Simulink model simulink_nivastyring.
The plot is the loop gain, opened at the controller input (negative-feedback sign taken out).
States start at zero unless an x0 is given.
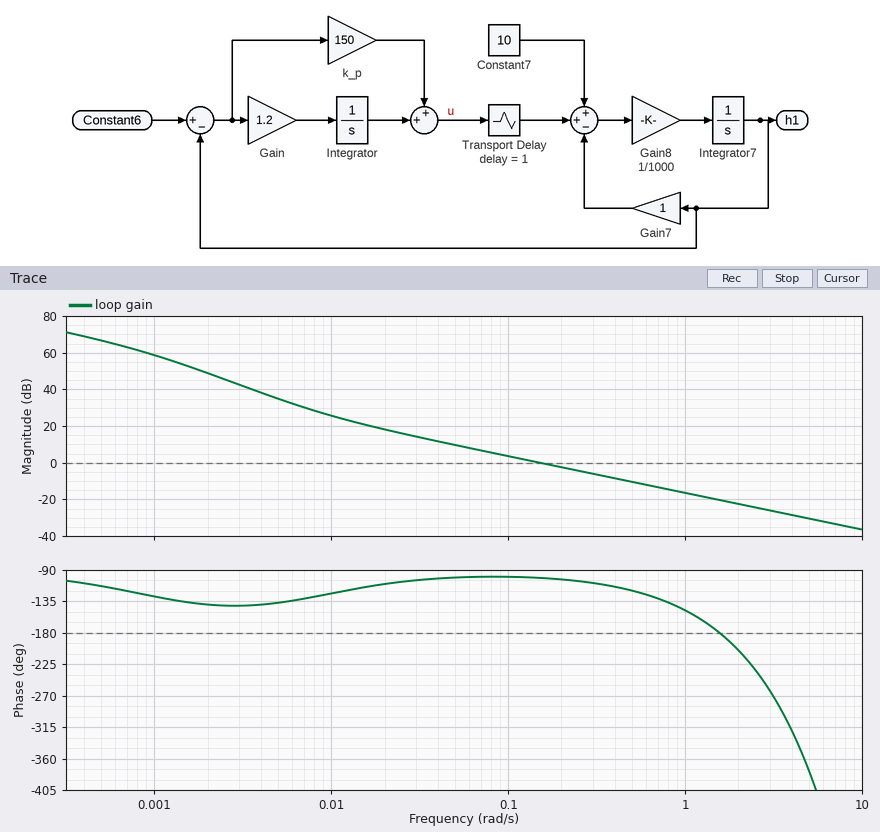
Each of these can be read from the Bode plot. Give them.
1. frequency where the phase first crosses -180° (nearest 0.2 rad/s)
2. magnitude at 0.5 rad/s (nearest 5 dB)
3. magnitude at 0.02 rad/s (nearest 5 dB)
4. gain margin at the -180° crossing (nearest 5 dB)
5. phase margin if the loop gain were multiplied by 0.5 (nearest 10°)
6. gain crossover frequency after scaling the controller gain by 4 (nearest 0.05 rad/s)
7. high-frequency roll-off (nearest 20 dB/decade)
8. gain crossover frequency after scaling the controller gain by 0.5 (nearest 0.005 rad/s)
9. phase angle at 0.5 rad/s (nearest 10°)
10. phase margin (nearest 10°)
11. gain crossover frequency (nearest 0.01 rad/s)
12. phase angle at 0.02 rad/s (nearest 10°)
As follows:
1.6 rad/s
-10 dB
20 dB
20 dB
80°
0.60 rad/s
-20 dB/decade
0.075 rad/s
-120°
80°
0.15 rad/s
-110°
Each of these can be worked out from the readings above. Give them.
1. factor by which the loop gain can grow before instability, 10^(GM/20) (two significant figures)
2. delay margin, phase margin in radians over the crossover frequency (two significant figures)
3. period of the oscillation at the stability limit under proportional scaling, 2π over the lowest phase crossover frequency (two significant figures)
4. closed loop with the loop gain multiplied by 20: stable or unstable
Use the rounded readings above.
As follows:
10
9.3 s
3.9 s
unstable
